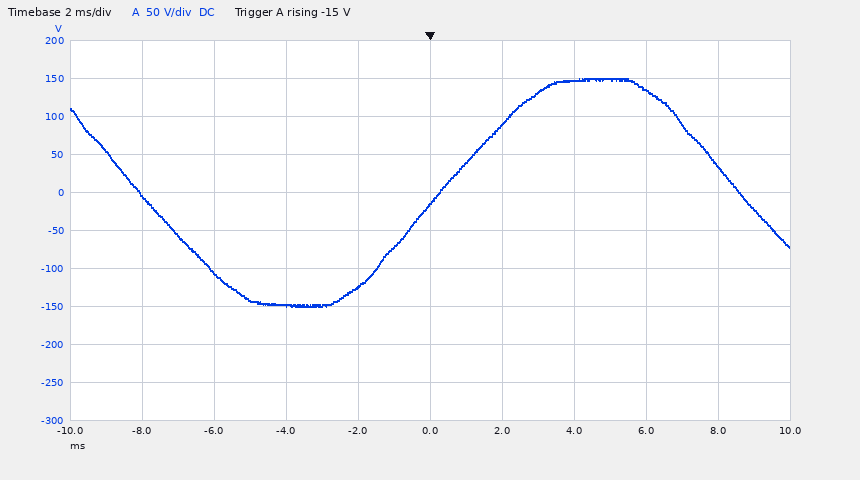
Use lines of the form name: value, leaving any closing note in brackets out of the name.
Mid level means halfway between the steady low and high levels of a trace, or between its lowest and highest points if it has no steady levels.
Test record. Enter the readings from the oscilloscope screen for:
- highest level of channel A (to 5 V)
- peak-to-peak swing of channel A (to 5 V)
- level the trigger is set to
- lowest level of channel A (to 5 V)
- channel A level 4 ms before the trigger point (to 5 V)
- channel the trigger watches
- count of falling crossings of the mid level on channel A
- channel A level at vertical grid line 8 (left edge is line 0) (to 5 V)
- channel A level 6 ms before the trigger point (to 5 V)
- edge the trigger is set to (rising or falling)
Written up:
highest level of channel A: 150 V
peak-to-peak swing of channel A: 300 V
level the trigger is set to: -15 V
lowest level of channel A: -150 V
channel A level 4 ms before the trigger point: -150 V
channel the trigger watches: channel A
count of falling crossings of the mid level on channel A: 2
channel A level at vertical grid line 8 (left edge is line 0): 135 V
channel A level 6 ms before the trigger point: -105 V
edge the trigger is set to: rising
